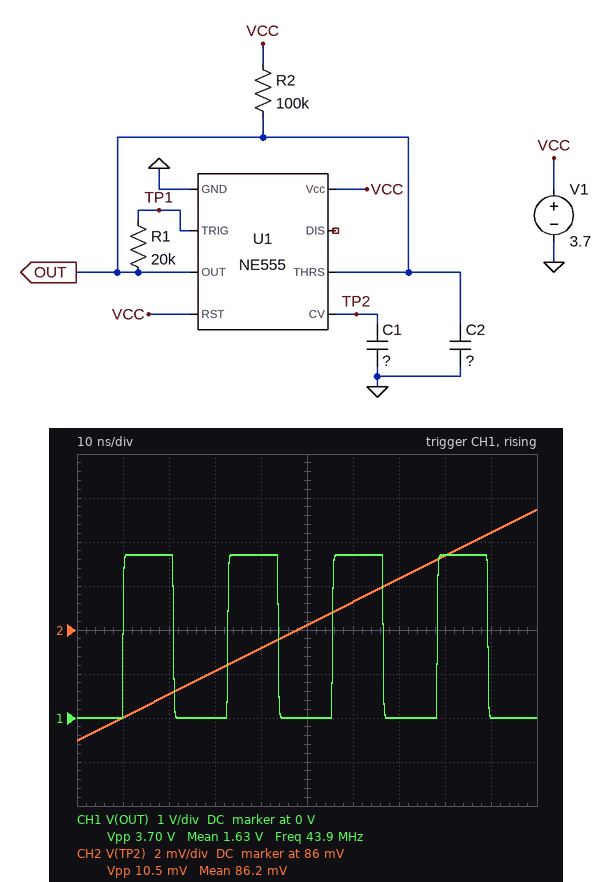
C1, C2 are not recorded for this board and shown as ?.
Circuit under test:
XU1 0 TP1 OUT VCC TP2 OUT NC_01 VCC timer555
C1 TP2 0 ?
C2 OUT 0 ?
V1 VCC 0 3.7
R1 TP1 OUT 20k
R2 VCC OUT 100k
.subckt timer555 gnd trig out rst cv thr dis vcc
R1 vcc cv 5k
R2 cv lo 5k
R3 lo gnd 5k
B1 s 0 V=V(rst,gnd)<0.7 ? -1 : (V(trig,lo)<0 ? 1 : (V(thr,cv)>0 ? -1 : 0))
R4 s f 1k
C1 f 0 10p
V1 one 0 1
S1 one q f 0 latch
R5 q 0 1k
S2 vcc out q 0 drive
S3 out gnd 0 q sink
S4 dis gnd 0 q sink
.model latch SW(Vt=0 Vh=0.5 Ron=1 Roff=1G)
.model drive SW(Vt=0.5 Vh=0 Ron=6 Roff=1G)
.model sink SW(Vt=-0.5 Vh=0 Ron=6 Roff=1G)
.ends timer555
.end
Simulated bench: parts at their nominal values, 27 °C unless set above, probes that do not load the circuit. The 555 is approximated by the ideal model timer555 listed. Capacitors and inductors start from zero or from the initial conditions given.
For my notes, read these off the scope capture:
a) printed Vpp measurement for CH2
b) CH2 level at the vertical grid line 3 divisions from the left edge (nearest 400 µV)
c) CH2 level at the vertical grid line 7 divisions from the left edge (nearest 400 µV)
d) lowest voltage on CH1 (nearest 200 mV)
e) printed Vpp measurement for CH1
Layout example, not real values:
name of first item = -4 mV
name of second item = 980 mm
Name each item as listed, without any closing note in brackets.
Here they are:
printed Vpp measurement for CH2 = 10.5 mV
CH2 level at the vertical grid line 3 divisions from the left edge = 84.0 mV
CH2 level at the vertical grid line 7 divisions from the left edge = 88.4 mV
lowest voltage on CH1 = 0 V
printed Vpp measurement for CH1 = 3.70 V
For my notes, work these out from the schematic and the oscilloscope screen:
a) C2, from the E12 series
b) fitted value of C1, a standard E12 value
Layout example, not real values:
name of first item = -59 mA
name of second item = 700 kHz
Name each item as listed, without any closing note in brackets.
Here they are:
C2, from the E12 series = 22 pF
fitted value of C1, a standard E12 value = 6.8 nF
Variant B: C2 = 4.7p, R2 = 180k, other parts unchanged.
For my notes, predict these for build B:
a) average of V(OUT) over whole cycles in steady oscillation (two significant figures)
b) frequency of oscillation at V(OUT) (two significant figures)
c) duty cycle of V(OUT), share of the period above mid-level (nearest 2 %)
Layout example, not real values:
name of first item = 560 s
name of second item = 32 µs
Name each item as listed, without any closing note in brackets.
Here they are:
average of V(OUT) over whole cycles in steady oscillation = 1.8 V
frequency of oscillation at V(OUT) = 45 MHz
duty cycle of V(OUT), share of the period above mid-level = 50 %
